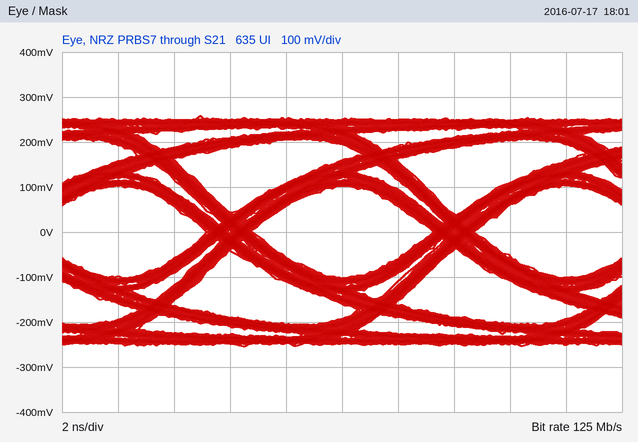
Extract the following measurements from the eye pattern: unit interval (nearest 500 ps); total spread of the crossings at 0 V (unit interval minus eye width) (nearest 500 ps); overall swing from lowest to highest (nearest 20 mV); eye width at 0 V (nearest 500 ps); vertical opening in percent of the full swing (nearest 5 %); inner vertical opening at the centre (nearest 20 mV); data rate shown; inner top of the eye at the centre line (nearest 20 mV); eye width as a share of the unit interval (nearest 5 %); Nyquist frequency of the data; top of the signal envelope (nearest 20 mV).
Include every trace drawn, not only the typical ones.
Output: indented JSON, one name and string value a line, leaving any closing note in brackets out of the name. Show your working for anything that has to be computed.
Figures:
{
  "unit interval": "8.0 ns",
  "total spread of the crossings at 0 V (unit interval minus eye width)": "1.5 ns",
  "overall swing from lowest to highest": "520 mV",
  "eye width at 0 V": "6.5 ns",
  "vertical opening in percent of the full swing": "200 mV / 520 mV ≈ 38.5 %, so 40 % to the nearest 5 %",
  "inner vertical opening at the centre": "200 mV",
  "data rate shown": "125 Mb/s",
  "inner top of the eye at the centre line": "100 mV",
  "eye width as a share of the unit interval": "6.5 ns / 8.0 ns ≈ 81.2 %, so 80 % to the nearest 5 %",
  "Nyquist frequency of the data": "62.5 MHz",
  "top of the signal envelope": "260 mV"
}
